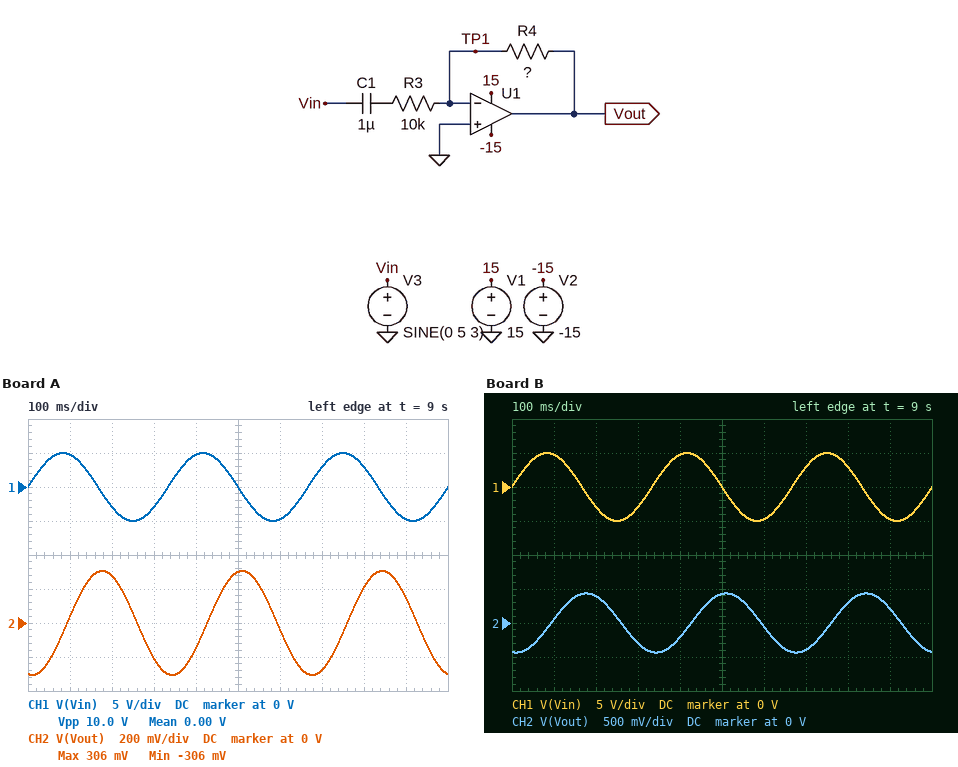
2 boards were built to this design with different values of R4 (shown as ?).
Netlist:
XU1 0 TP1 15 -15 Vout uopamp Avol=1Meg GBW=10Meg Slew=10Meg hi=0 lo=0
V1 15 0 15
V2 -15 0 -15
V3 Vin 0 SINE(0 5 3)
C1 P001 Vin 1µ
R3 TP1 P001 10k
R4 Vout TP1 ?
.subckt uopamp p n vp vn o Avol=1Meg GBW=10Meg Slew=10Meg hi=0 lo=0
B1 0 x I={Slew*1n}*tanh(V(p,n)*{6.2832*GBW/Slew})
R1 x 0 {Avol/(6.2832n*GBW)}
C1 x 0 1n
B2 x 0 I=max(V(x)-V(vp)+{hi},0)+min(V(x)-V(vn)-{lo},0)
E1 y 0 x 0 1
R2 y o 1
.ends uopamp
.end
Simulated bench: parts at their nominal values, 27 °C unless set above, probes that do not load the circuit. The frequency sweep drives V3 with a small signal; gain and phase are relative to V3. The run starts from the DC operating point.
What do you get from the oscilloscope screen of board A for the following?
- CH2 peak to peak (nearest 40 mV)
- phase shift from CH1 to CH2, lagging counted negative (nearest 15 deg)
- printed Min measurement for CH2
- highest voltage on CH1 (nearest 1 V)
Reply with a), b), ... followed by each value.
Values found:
a) 600 mV
b) -105 deg
c) -306 mV
d) 5 V
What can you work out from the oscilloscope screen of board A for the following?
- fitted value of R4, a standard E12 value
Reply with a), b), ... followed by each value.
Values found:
a) 3.3 kΩ
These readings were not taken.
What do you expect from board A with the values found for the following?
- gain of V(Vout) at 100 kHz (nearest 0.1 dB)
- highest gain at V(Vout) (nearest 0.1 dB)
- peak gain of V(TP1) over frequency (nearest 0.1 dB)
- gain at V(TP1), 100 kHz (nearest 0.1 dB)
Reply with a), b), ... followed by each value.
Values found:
a) -9.6 dB
b) -9.6 dB
c) -12.1 dB
d) -49.6 dB
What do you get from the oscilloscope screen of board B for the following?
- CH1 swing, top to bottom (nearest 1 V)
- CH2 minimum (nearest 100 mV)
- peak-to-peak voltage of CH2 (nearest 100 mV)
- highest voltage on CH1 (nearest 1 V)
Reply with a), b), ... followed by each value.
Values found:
a) 10 V
b) -400 mV
c) 900 mV
d) 5 V
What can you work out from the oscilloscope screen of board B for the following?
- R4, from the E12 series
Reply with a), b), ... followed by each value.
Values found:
a) 4.7 kΩ
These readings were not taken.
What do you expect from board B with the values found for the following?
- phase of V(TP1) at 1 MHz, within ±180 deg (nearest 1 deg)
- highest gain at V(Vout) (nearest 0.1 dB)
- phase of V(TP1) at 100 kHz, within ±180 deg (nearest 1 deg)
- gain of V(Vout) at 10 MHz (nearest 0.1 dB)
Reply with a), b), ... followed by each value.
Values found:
a) 82 deg
b) -6.6 dB
c) 89 deg
d) -11.6 dB
